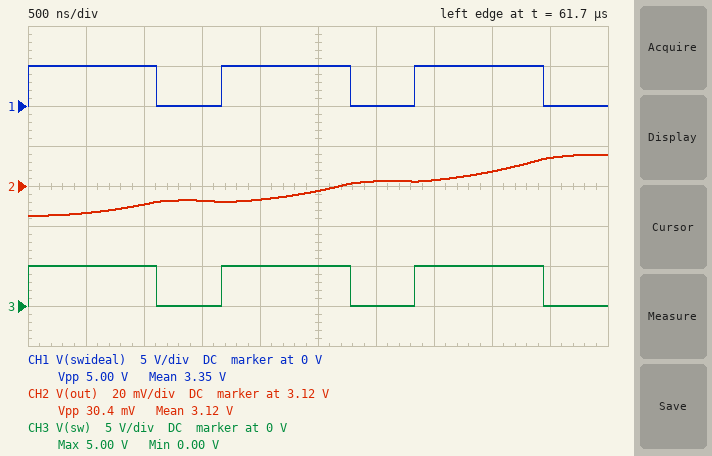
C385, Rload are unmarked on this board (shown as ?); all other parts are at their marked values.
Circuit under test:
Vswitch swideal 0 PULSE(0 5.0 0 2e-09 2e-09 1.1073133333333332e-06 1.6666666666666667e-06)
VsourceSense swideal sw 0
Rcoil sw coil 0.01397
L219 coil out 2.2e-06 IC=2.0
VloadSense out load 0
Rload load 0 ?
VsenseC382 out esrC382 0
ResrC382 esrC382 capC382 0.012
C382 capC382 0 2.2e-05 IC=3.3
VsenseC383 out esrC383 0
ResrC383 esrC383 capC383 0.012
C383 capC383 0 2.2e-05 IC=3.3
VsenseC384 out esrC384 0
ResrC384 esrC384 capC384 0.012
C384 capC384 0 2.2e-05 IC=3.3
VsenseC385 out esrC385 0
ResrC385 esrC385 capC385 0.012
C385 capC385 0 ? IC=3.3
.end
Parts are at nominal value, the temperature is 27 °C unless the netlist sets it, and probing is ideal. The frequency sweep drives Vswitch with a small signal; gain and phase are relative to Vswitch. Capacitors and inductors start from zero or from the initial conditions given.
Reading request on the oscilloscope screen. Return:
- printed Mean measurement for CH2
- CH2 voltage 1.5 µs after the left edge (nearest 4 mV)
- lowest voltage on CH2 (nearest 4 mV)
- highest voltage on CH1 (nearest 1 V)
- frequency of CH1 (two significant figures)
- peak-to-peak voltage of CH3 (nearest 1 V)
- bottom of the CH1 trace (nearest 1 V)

3.12 V
3.112 V
3.104 V
5 V
600 kHz
5 V
0 V
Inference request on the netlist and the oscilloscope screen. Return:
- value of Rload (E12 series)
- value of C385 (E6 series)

4.7 Ω
6.8 µF
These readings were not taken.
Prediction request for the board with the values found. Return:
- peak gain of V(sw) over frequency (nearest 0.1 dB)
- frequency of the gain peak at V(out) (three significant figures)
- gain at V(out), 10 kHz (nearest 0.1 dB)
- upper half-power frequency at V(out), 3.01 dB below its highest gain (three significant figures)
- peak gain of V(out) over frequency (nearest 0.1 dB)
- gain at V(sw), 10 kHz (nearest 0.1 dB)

0 dB
12.5 kHz
8.3 dB
13.4 kHz
17.3 dB
0 dB
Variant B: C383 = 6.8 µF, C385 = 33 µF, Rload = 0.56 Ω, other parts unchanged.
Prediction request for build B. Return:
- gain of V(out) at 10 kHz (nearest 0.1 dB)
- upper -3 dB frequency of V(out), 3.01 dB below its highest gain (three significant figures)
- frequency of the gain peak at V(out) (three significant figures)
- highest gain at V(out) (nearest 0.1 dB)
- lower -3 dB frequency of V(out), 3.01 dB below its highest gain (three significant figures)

7.0 dB
13.5 kHz
11.4 kHz
8.1 dB
8.68 kHz
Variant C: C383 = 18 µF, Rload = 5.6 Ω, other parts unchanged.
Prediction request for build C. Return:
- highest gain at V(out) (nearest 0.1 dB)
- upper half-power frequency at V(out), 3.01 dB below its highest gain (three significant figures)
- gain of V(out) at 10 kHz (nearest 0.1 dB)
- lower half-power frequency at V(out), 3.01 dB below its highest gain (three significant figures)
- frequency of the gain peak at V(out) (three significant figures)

17.8 dB
13.7 kHz
7.6 dB
12.0 kHz
12.9 kHz
